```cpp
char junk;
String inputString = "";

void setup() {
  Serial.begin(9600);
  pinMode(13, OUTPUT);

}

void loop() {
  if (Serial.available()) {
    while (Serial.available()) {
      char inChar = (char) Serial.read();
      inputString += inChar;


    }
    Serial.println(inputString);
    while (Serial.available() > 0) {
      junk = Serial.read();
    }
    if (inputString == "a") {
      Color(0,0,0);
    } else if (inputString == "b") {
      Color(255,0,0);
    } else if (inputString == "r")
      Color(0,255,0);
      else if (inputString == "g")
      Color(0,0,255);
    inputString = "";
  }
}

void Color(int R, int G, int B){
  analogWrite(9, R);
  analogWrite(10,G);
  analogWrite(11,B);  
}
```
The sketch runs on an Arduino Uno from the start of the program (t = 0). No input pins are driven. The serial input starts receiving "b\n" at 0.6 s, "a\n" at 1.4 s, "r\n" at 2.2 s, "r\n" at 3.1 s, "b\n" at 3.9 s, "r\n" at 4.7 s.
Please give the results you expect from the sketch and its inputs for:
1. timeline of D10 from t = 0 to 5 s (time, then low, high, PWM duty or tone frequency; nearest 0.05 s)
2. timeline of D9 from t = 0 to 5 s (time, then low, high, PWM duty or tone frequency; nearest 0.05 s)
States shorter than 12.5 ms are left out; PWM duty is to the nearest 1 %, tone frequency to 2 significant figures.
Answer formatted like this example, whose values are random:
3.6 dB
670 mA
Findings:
0.6 s low; 2.2 s high; 3.9 s low; 4.7 s high
0.6 s high; 1.4 s low; 3.9 s high; 4.7 s low
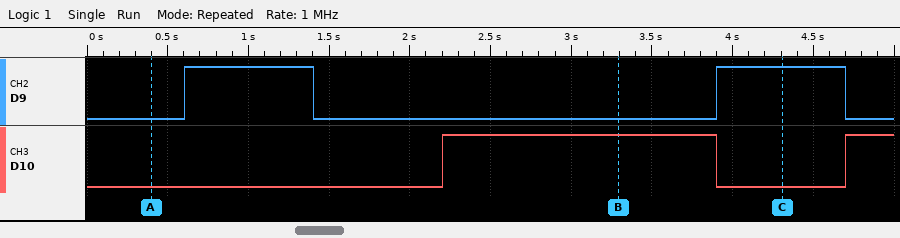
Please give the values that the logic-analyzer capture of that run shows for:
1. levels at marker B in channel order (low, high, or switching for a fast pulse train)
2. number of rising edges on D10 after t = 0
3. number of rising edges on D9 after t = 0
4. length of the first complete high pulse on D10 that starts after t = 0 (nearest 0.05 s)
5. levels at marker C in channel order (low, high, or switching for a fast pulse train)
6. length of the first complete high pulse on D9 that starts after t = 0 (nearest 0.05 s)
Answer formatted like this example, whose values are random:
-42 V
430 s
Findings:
D9 low, D10 high
2
2
1.70 s
D9 high, D10 low
0.80 s
